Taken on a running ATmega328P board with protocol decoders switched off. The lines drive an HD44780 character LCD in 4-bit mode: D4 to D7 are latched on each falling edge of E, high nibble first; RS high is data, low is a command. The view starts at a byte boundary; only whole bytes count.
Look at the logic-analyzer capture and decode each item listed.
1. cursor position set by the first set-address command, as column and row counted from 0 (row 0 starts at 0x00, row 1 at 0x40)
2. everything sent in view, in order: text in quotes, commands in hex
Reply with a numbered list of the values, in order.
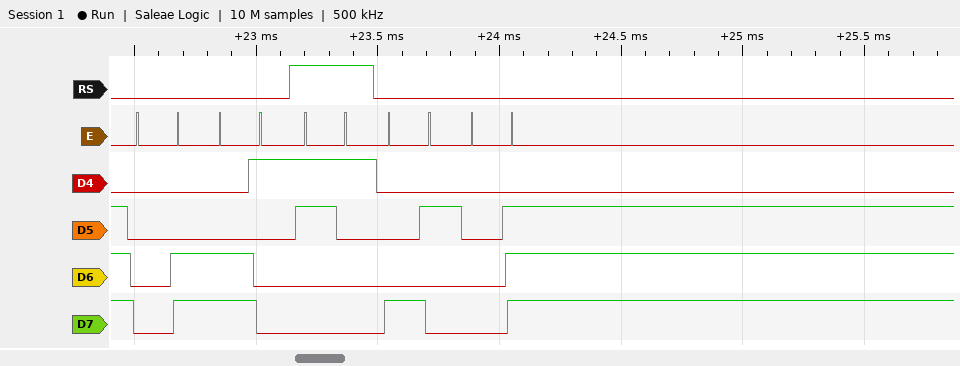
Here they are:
1. column 1, row 1
2. 0x0C 0xC1 "1" 0x82 0x0E
